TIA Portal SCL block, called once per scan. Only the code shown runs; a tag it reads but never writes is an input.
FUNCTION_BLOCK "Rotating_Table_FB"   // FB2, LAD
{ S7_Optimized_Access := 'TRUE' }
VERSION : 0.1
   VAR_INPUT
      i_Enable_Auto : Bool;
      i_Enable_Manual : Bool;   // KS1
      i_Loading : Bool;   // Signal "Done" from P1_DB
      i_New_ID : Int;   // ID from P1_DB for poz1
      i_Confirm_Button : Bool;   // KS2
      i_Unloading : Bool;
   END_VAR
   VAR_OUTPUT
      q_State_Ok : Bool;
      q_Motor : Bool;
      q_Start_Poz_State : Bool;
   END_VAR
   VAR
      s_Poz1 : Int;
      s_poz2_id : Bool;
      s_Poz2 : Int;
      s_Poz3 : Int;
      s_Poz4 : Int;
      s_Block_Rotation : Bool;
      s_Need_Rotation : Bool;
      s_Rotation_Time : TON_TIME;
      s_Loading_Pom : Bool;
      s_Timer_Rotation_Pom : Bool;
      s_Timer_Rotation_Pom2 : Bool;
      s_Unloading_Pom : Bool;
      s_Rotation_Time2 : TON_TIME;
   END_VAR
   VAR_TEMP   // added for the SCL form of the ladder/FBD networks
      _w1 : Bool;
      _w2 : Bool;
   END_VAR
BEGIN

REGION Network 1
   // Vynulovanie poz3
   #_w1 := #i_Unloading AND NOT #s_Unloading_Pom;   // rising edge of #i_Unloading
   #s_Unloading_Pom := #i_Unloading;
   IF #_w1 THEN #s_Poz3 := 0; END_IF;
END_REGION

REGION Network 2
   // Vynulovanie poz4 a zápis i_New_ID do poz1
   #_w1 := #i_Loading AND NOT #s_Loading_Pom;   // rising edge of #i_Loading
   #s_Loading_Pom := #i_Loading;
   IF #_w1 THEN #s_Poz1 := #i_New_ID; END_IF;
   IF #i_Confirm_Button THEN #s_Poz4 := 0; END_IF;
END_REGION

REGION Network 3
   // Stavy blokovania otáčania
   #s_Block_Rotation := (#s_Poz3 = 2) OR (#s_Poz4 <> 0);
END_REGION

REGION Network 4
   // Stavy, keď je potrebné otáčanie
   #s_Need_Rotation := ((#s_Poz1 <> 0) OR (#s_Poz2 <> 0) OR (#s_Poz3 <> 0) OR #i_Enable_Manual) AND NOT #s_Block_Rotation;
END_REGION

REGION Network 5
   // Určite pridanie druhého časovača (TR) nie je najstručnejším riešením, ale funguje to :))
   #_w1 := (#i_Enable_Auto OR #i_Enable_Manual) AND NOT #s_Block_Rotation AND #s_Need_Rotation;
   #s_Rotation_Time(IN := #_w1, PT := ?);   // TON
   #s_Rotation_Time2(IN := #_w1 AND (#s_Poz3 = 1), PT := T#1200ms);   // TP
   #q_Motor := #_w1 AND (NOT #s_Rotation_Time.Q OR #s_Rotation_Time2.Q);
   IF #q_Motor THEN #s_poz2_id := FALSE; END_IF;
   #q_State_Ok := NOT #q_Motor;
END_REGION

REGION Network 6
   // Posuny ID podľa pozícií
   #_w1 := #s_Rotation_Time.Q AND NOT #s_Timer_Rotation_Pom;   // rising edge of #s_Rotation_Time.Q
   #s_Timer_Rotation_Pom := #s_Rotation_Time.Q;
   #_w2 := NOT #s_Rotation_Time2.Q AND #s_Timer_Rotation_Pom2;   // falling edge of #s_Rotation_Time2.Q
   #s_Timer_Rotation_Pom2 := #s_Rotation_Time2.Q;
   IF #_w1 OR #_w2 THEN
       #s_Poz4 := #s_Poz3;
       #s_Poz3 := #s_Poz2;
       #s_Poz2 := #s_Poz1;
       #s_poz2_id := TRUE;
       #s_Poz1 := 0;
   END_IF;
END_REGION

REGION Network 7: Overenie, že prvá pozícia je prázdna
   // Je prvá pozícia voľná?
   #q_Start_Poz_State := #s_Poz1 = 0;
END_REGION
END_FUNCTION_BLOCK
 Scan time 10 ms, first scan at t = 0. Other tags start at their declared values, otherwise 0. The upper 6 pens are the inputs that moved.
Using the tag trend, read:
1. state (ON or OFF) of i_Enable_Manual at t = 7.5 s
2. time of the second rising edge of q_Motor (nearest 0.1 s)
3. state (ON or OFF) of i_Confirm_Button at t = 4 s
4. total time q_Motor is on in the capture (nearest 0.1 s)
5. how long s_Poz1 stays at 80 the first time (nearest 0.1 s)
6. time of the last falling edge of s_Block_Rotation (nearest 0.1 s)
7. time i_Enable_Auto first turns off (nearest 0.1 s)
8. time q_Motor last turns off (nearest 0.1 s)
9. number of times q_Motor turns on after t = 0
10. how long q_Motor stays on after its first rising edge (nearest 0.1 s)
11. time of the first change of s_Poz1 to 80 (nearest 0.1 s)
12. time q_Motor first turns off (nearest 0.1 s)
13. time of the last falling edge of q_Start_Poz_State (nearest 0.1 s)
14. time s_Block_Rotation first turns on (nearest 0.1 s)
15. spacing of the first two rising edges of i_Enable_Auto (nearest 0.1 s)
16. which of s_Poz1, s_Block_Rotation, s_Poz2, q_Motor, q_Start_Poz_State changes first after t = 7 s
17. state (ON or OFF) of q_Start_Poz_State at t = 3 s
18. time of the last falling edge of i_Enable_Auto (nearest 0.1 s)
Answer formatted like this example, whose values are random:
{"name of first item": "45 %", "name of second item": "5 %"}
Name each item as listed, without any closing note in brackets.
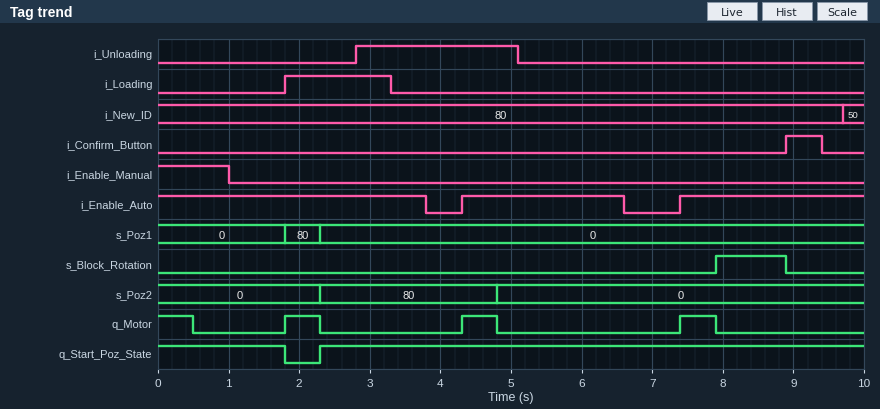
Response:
{"state (ON or OFF) of i_Enable_Manual at t = 7.5 s": "OFF", "time of the second rising edge of q_Motor": "4.3 s", "state (ON or OFF) of i_Confirm_Button at t = 4 s": "OFF", "total time q_Motor is on in the capture": "2.0 s", "how long s_Poz1 stays at 80 the first time": "0.5 s", "time of the last falling edge of s_Block_Rotation": "8.9 s", "time i_Enable_Auto first turns off": "3.8 s", "time q_Motor last turns off": "7.9 s", "number of times q_Motor turns on after t = 0": "3", "how long q_Motor stays on after its first rising edge": "0.5 s", "time of the first change of s_Poz1 to 80": "1.8 s", "time q_Motor first turns off": "0.5 s", "time of the last falling edge of q_Start_Poz_State": "1.8 s", "time s_Block_Rotation first turns on": "7.9 s", "spacing of the first two rising edges of i_Enable_Auto": "3.1 s", "which of s_Poz1, s_Block_Rotation, s_Poz2, q_Motor, q_Start_Poz_State changes first after t = 7 s": "q_Motor", "state (ON or OFF) of q_Start_Poz_State at t = 3 s": "ON", "time of the last falling edge of i_Enable_Auto": "6.6 s"}
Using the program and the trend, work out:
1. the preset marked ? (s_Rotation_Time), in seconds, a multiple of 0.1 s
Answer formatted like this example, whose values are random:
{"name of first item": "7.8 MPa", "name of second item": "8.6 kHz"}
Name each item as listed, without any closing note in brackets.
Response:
{"the preset marked ? (s_Rotation_Time), in seconds, a multiple of 0.1 s": "0.5 s"}
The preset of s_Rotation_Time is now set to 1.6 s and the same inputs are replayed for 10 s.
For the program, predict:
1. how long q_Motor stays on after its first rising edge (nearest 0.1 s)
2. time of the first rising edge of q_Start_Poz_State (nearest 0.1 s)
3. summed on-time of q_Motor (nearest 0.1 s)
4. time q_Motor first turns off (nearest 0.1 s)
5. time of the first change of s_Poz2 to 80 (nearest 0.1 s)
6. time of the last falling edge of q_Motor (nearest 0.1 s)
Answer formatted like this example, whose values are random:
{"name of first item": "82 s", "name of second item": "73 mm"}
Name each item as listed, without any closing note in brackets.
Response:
{"how long q_Motor stays on after its first rising edge": "1.6 s", "time of the first rising edge of q_Start_Poz_State": "3.4 s", "summed on-time of q_Motor": "5.8 s", "time q_Motor first turns off": "1.0 s", "time of the first change of s_Poz2 to 80": "3.4 s", "time of the last falling edge of q_Motor": "9.0 s"}
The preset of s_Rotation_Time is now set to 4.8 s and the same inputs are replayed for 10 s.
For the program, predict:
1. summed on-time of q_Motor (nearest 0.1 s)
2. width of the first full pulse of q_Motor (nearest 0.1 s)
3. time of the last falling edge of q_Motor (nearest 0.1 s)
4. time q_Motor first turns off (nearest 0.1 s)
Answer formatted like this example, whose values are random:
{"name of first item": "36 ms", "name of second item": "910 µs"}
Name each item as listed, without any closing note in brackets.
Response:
{"summed on-time of q_Motor": "7.9 s", "width of the first full pulse of q_Motor": "2.0 s", "time of the last falling edge of q_Motor": "6.6 s", "time q_Motor first turns off": "1.0 s"}
